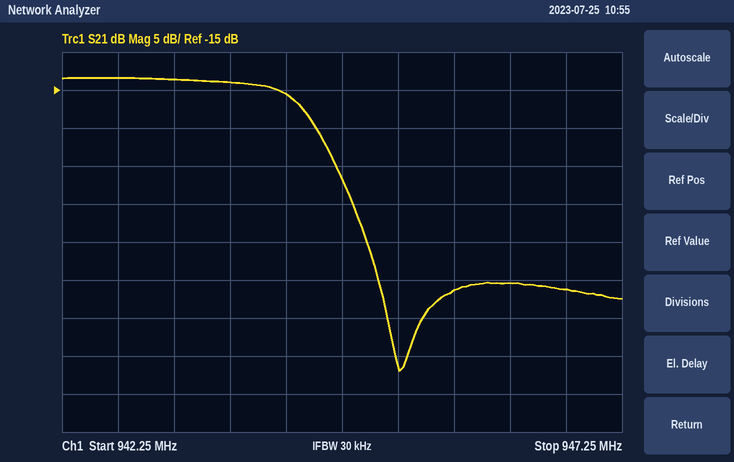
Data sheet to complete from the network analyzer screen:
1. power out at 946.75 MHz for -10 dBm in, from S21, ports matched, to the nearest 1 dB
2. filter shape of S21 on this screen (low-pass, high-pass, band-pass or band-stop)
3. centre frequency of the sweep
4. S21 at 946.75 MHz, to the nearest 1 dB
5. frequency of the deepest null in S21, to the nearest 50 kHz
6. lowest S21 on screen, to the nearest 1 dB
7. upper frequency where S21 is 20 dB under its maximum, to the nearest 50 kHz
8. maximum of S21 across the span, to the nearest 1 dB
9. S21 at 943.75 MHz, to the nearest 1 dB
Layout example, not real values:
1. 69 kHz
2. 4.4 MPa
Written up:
1. -51 dBm
2. low-pass
3. 944.75 MHz
4. -41 dB
5. 945.25 MHz
6. -52 dB
7. 944.95 MHz
8. -13 dB
9. -14 dB
